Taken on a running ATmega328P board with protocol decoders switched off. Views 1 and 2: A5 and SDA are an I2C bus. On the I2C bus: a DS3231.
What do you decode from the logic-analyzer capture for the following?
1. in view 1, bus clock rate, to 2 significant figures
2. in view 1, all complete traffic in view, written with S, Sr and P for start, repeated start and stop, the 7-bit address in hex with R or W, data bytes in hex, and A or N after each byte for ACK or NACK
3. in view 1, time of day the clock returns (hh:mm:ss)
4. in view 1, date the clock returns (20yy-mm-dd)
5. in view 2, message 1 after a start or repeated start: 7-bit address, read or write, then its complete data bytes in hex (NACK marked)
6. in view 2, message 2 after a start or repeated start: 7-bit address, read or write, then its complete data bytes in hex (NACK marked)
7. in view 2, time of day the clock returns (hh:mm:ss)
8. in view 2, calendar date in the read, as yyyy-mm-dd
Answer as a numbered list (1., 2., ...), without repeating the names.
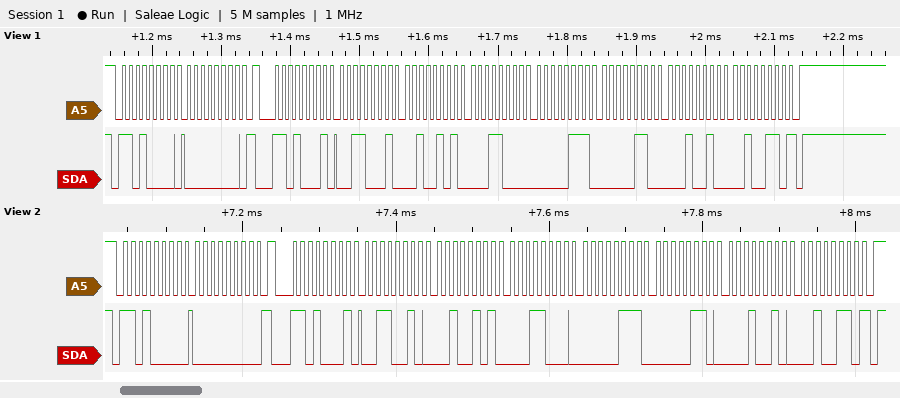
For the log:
1. 100 kHz
2. S 68W A 00 A Sr 68R A 31 A 25 A 18 A 07 A 06 A 12 A 26 N P
3. 18:25:31
4. 2026-12-06
5. 0x68 write: 00
6. 0x68 read: 32 25 18 07 06 12 26 NACK
7. 18:25:32
8. 2026-12-06
